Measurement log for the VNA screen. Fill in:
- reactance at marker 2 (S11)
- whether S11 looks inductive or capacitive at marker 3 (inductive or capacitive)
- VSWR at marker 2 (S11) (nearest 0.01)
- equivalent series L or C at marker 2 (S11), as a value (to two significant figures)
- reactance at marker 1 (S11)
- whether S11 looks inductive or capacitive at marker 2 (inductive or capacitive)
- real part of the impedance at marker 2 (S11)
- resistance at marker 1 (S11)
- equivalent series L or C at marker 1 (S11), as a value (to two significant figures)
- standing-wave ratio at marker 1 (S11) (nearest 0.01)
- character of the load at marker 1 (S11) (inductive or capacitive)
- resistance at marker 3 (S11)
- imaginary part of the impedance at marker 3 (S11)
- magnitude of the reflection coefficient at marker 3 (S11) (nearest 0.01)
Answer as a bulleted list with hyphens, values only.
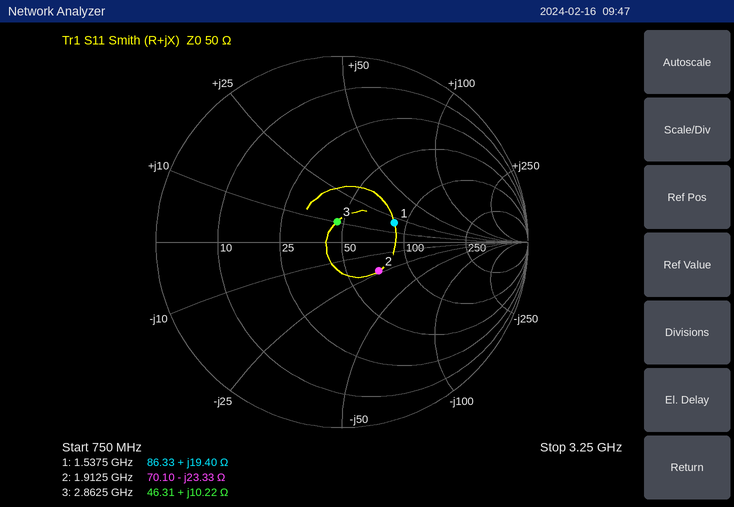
- -23.33 Ω
- inductive
- 1.67
- 3.6 pF
- +19.40 Ω
- capacitive
- 70.10 Ω
- 86.33 Ω
- 2.0 nH
- 1.85
- inductive
- 46.31 Ω
- +10.22 Ω
- 0.11
